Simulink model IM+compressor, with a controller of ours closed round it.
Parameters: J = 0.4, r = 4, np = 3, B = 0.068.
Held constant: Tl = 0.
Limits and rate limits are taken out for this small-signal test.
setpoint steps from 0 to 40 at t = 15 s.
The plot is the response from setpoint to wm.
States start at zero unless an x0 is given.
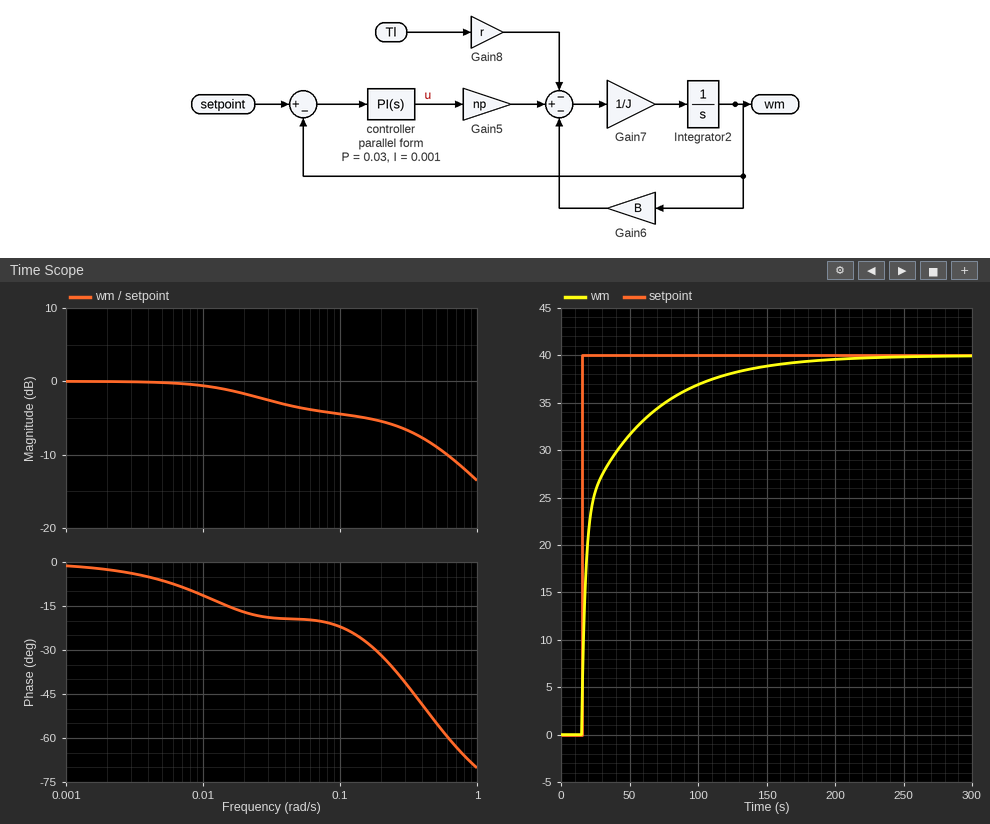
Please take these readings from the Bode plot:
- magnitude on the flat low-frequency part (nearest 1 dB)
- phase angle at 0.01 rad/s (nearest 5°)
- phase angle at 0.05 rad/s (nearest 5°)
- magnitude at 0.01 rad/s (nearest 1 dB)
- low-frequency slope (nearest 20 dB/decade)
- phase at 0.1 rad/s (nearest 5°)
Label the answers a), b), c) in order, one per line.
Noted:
a) 0 dB
b) -10°
c) -20°
d) -1 dB
e) 0 dB/decade
f) -20°
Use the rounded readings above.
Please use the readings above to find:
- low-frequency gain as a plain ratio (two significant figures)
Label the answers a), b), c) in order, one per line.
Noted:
a) 1.0
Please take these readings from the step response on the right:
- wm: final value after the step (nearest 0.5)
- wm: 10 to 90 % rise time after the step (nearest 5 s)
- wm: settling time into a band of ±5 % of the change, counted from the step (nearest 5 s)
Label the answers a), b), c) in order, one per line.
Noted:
a) 40.0
b) 70 s
c) 105 s
